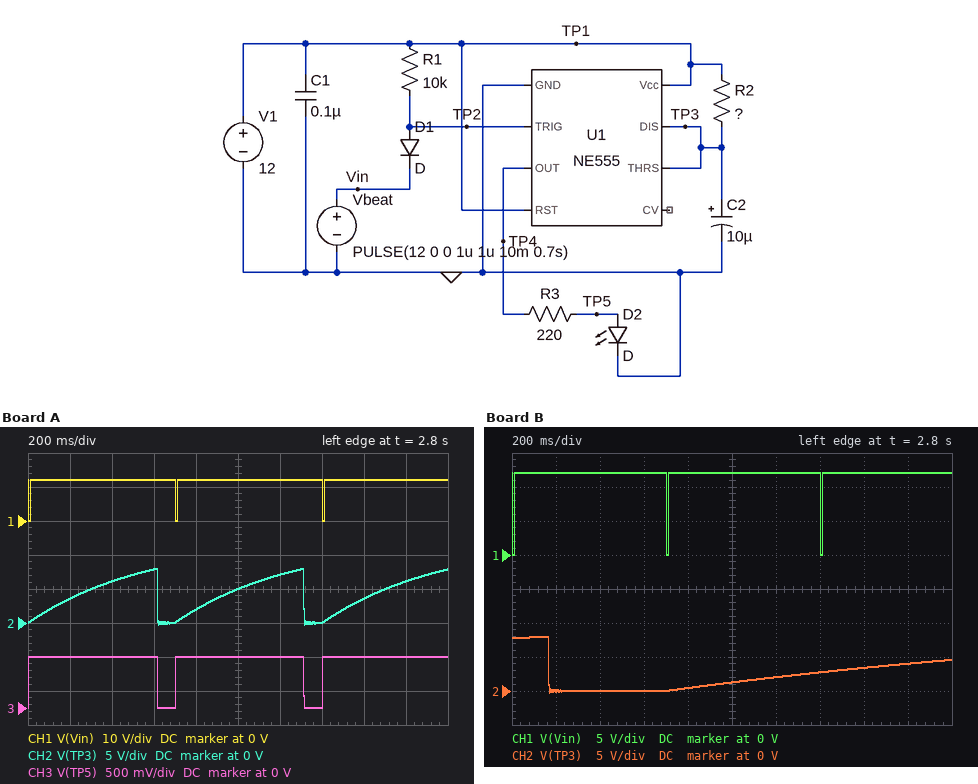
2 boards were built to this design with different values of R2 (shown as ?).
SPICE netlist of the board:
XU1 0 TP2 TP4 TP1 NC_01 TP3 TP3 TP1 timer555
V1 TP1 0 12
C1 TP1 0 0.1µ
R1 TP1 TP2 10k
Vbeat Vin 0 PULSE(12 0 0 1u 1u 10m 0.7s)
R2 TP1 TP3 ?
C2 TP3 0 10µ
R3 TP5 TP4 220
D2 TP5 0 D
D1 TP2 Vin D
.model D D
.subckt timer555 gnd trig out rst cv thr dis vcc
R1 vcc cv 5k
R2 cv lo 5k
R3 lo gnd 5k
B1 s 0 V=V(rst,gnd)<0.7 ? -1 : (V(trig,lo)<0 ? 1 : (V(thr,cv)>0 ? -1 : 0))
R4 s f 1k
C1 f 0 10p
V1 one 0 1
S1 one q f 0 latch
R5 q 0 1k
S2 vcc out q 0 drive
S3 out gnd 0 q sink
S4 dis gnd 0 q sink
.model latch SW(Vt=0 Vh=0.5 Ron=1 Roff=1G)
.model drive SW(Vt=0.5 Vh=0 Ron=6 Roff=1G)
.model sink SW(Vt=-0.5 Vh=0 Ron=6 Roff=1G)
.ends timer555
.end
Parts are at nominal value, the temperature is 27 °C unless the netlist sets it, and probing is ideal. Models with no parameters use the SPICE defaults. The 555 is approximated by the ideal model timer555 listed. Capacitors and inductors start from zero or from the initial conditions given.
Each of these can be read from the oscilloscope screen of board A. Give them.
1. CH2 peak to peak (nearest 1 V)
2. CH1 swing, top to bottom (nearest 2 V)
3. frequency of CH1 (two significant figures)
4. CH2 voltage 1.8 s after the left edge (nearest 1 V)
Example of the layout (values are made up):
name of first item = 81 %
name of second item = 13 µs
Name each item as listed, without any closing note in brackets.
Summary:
CH2 peak to peak = 8 V
CH1 swing, top to bottom = 12 V
frequency of CH1 = 1.4 Hz
CH2 voltage 1.8 s after the left edge = 6 V
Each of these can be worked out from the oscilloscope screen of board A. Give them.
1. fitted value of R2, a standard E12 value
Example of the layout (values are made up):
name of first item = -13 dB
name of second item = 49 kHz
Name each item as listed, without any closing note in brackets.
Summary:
fitted value of R2, a standard E12 value = 56 kΩ
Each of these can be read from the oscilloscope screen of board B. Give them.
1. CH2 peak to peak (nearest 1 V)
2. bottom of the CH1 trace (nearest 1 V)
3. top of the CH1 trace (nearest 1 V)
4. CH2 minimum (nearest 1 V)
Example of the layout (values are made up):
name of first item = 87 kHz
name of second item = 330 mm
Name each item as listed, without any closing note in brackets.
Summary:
CH2 peak to peak = 8 V
bottom of the CH1 trace = 0 V
top of the CH1 trace = 12 V
CH2 minimum = 0 V
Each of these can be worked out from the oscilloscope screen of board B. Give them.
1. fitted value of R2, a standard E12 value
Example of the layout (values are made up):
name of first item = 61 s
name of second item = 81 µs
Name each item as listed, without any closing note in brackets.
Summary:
fitted value of R2, a standard E12 value = 270 kΩ
